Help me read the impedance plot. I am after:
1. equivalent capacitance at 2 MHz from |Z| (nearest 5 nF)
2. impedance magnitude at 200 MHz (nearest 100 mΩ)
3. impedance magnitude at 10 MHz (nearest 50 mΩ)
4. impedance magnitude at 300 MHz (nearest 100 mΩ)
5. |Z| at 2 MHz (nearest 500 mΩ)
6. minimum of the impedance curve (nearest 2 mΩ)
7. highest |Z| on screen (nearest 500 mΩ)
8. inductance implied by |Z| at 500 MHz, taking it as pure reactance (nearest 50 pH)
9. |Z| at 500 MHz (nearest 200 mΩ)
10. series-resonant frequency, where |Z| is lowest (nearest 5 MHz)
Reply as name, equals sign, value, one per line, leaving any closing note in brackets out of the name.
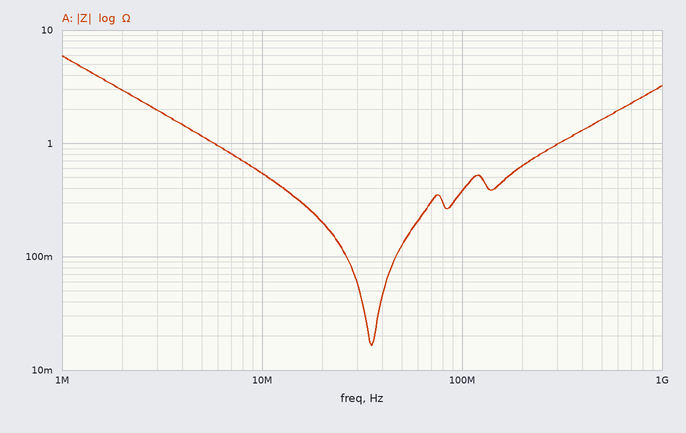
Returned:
equivalent capacitance at 2 MHz from |Z| = 25 nF
impedance magnitude at 200 MHz = 600 mΩ
impedance magnitude at 10 MHz = 550 mΩ
impedance magnitude at 300 MHz = 1.0 Ω
|Z| at 2 MHz = 3.0 Ω
minimum of the impedance curve = 16 mΩ
highest |Z| on screen = 6.0 Ω
inductance implied by |Z| at 500 MHz, taking it as pure reactance = 500 pH
|Z| at 500 MHz = 1.6 Ω
series-resonant frequency, where |Z| is lowest = 35 MHz
